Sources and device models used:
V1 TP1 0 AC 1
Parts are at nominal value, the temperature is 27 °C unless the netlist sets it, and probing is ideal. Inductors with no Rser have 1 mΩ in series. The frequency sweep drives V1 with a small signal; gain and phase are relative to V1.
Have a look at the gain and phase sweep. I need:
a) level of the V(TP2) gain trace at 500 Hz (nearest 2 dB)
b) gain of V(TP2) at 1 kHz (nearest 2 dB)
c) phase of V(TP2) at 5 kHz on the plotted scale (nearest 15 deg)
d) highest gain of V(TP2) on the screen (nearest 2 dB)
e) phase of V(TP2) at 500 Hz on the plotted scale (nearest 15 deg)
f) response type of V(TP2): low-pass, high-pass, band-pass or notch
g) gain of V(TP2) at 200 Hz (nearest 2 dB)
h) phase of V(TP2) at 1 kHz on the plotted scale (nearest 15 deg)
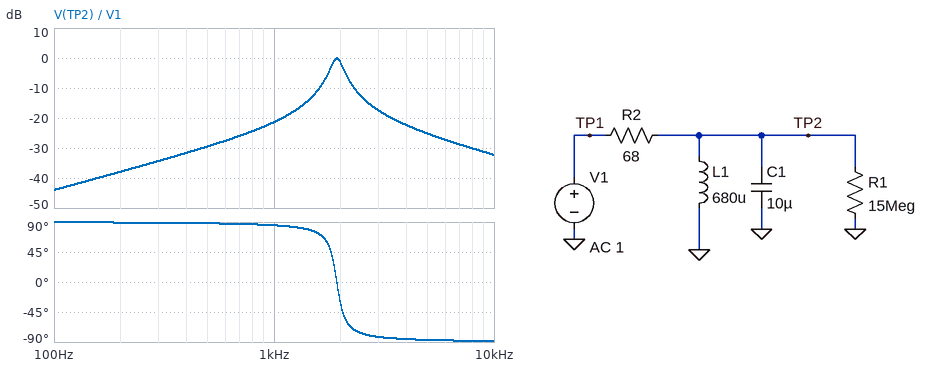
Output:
-30 dB
-22 dB
-90 deg
0 dB
90 deg
band-pass
-38 dB
90 deg
